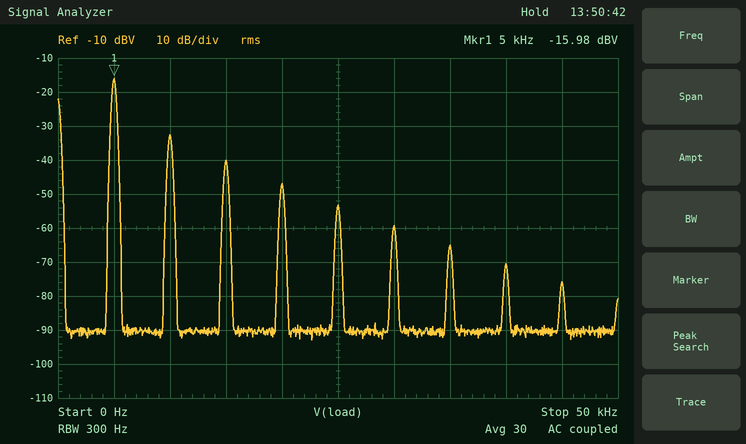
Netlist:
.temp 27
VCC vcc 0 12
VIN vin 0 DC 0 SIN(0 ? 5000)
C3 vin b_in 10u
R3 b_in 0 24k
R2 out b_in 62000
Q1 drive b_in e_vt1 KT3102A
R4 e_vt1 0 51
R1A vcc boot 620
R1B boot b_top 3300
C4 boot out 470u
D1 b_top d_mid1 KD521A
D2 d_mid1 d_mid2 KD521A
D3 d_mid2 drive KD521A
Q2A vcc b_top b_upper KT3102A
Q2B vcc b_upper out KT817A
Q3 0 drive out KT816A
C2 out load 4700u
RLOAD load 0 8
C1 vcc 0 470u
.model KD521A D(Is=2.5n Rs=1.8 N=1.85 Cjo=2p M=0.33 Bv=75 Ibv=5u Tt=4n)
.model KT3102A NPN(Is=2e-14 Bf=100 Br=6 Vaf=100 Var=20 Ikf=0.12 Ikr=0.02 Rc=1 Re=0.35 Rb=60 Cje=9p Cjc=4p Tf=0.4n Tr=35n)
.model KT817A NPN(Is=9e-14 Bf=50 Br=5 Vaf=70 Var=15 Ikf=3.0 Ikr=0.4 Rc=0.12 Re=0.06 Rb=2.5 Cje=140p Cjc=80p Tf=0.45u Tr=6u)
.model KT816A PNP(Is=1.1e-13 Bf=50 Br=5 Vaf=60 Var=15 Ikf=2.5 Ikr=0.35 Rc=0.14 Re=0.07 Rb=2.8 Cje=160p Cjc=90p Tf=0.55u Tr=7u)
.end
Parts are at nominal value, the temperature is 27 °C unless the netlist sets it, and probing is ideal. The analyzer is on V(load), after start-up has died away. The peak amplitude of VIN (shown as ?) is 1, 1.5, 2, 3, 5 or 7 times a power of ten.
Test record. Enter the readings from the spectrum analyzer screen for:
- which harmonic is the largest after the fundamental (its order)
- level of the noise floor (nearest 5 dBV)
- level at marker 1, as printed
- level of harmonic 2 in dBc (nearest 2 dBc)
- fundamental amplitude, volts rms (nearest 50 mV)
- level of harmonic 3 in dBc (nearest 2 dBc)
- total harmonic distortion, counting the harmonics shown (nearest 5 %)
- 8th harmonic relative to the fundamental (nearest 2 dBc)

2
-90 dBV
-15.98 dBV
-16 dBc
150 mV
-24 dBc
15 %
-54 dBc
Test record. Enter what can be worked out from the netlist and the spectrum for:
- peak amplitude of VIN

30 mV
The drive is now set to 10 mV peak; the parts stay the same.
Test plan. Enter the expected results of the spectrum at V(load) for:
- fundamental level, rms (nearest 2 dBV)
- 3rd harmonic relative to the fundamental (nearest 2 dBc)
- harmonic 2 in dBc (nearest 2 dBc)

-26 dBV
-48 dBc
-30 dBc
